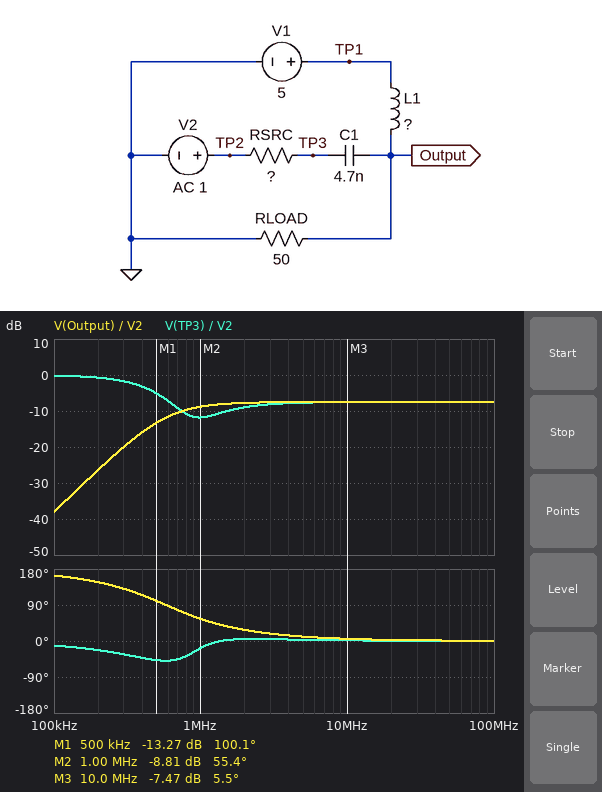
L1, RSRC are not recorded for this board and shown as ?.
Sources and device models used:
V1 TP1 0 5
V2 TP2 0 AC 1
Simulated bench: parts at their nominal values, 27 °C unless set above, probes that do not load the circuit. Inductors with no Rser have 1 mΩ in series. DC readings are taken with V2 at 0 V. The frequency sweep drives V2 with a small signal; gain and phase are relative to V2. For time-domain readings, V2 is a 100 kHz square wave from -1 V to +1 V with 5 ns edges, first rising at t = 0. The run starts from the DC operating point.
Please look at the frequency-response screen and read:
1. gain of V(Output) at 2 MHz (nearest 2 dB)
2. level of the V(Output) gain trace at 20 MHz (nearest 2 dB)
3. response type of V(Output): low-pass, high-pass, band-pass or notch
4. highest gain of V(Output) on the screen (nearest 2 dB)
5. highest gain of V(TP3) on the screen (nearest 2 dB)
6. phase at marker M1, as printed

-8 dB
-8 dB
high-pass
-8 dB
0 dB
100.1 deg
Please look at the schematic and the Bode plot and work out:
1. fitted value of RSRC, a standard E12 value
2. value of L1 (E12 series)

68 Ω
6.8 µH
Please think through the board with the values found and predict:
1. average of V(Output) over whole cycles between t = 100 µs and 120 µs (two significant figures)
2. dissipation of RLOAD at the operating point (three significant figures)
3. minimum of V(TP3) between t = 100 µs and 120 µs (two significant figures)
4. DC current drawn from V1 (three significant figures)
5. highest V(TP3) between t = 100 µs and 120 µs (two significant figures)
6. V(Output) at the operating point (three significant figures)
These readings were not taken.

5.0 V
500 mW
-1.0 V
100 mA
1.0 V
5.00 V
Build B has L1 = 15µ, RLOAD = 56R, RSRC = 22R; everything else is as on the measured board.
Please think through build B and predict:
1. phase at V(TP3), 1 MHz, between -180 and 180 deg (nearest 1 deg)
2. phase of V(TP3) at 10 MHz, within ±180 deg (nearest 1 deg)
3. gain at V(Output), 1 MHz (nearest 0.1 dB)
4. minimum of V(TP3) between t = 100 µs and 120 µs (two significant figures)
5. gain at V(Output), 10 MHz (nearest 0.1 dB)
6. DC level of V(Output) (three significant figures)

-4 deg
0 deg
-2.5 dB
-1.1 V
-2.9 dB
5.00 V
